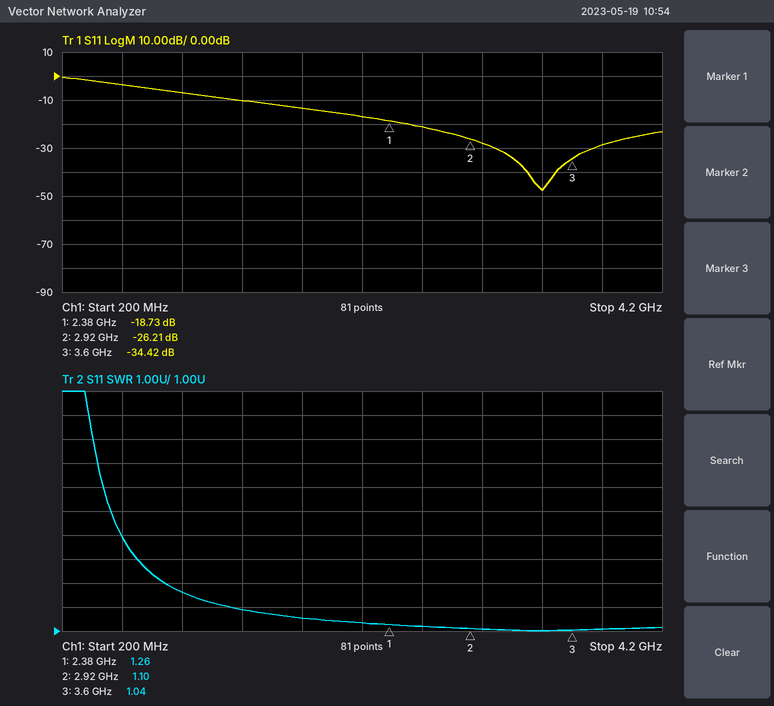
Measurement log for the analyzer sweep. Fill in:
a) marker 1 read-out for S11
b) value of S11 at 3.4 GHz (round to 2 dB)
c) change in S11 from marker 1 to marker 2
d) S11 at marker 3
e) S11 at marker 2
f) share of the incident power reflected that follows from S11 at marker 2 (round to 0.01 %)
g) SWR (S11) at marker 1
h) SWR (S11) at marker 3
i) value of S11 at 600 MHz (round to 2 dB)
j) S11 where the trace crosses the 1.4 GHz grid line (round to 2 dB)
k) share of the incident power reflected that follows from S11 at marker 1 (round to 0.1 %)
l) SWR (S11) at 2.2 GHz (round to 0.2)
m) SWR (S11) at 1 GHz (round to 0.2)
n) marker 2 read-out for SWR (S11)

-18.73 dB
-48 dB
-7.48 dB
-34.42 dB
-26.21 dB
0.24 %
1.26
1.04
-4 dB
-10 dB
1.3 %
1.4
2.6
1.10
